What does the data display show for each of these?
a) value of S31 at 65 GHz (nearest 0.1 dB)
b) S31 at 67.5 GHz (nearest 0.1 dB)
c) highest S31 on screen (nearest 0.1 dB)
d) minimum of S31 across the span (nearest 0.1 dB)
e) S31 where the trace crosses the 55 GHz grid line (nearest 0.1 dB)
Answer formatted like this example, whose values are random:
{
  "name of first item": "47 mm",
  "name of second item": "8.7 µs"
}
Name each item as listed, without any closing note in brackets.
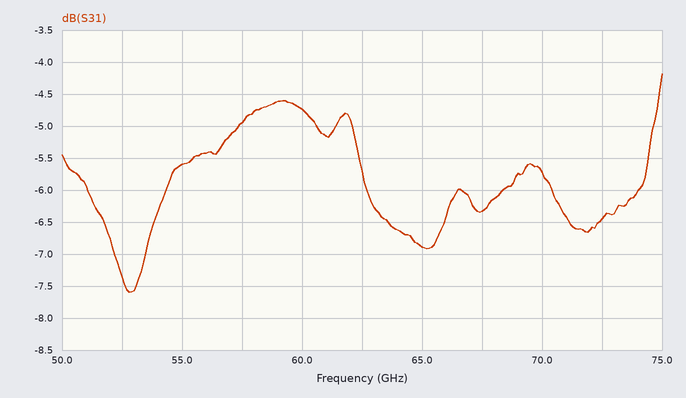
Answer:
{
  "value of S31 at 65 GHz": "-6.9 dB",
  "S31 at 67.5 GHz": "-6.3 dB",
  "highest S31 on screen": "-4.2 dB",
  "minimum of S31 across the span": "-7.6 dB",
  "S31 where the trace crosses the 55 GHz grid line": "-5.6 dB"
}
